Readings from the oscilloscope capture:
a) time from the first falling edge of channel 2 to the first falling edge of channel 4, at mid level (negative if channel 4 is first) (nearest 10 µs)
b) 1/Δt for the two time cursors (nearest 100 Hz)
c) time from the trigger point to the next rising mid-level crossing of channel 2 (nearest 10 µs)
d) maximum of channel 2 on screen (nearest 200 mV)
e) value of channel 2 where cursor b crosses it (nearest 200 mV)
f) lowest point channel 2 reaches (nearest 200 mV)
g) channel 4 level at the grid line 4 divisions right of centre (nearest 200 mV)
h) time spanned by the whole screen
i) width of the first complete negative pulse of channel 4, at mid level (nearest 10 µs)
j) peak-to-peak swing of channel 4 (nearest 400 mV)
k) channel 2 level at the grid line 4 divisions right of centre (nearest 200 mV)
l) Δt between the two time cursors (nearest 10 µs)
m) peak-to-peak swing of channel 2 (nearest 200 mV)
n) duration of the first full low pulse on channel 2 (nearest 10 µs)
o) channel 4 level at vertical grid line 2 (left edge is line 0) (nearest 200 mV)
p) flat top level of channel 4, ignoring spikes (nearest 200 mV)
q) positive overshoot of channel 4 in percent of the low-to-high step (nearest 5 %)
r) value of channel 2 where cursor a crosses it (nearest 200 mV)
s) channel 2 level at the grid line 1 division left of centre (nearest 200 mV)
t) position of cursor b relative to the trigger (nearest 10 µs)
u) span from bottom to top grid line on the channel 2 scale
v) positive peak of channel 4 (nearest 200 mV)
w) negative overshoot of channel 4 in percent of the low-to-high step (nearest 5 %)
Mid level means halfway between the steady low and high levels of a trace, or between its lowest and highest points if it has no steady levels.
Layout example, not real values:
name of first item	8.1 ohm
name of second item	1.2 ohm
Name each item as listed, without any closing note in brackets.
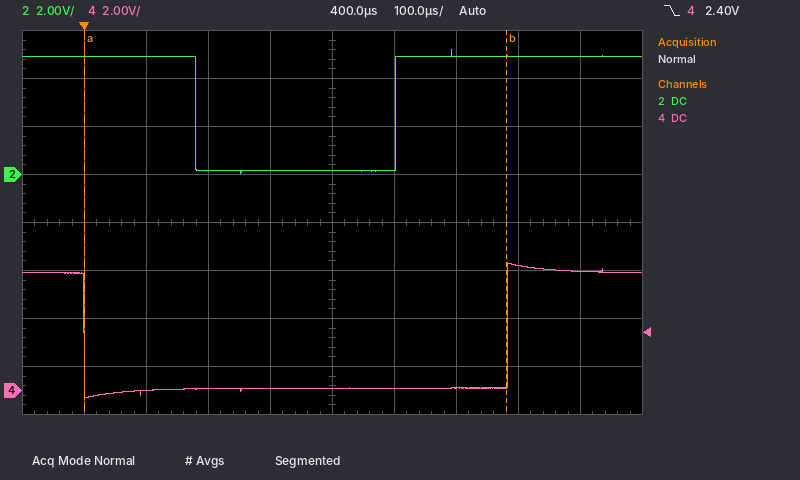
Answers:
time from the first falling edge of channel 2 to the first falling edge of channel 4, at mid level (negative if channel 4 is first)	-180 µs
1/Δt for the two time cursors	1.5 kHz
time from the trigger point to the next rising mid-level crossing of channel 2	500 µs
maximum of channel 2 on screen	5.2 V
value of channel 2 where cursor b crosses it	5.0 V
lowest point channel 2 reaches	0.0 V
channel 4 level at the grid line 4 divisions right of centre	5.0 V
time spanned by the whole screen	1 ms
width of the first complete negative pulse of channel 4, at mid level	680 µs
peak-to-peak swing of channel 4	5.6 V
channel 2 level at the grid line 4 divisions right of centre	5.0 V
Δt between the two time cursors	680 µs
peak-to-peak swing of channel 2	5.2 V
duration of the first full low pulse on channel 2	320 µs
channel 4 level at vertical grid line 2 (left edge is line 0)	0.0 V
flat top level of channel 4, ignoring spikes	5.0 V
positive overshoot of channel 4 in percent of the low-to-high step	10 %
value of channel 2 where cursor a crosses it	5.0 V
channel 2 level at the grid line 1 division left of centre	200 mV
position of cursor b relative to the trigger	+680 µs
span from bottom to top grid line on the channel 2 scale	16 V
positive peak of channel 4	5.4 V
negative overshoot of channel 4 in percent of the low-to-high step	10 %
